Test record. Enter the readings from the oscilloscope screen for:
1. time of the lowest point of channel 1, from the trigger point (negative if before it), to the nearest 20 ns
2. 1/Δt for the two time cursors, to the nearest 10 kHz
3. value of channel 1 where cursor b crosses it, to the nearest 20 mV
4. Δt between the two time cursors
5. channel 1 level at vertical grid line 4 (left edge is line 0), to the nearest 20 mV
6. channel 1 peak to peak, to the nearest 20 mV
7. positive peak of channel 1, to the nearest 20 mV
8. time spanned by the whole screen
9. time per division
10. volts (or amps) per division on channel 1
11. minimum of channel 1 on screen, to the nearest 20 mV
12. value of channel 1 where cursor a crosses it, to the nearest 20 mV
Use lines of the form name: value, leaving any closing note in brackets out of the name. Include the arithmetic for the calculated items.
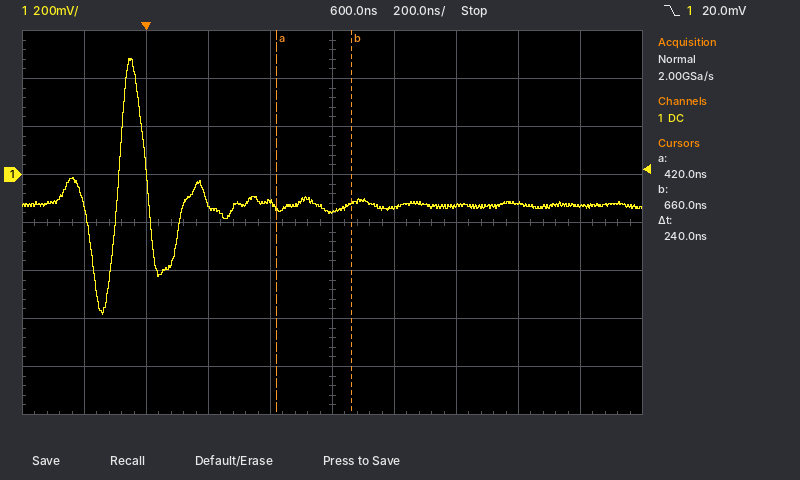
time of the lowest point of channel 1, from the trigger point (negative if before it), to the nearest 20 ns: -140 ns
1/Δt for the two time cursors, to the nearest 10 kHz: 1 / 240 ns ≈ 4.17 MHz
value of channel 1 where cursor b crosses it, to the nearest 20 mV: -120 mV
Δt between the two time cursors: 240 ns
channel 1 level at vertical grid line 4 (left edge is line 0), to the nearest 20 mV: -120 mV
channel 1 peak to peak, to the nearest 20 mV: 480 mV − (-580 mV) = 1.06 V
positive peak of channel 1, to the nearest 20 mV: 480 mV
time spanned by the whole screen: 2 µs
time per division: 200 ns
volts (or amps) per division on channel 1: 200 mV
minimum of channel 1 on screen, to the nearest 20 mV: -580 mV
value of channel 1 where cursor a crosses it, to the nearest 20 mV: -140 mV
